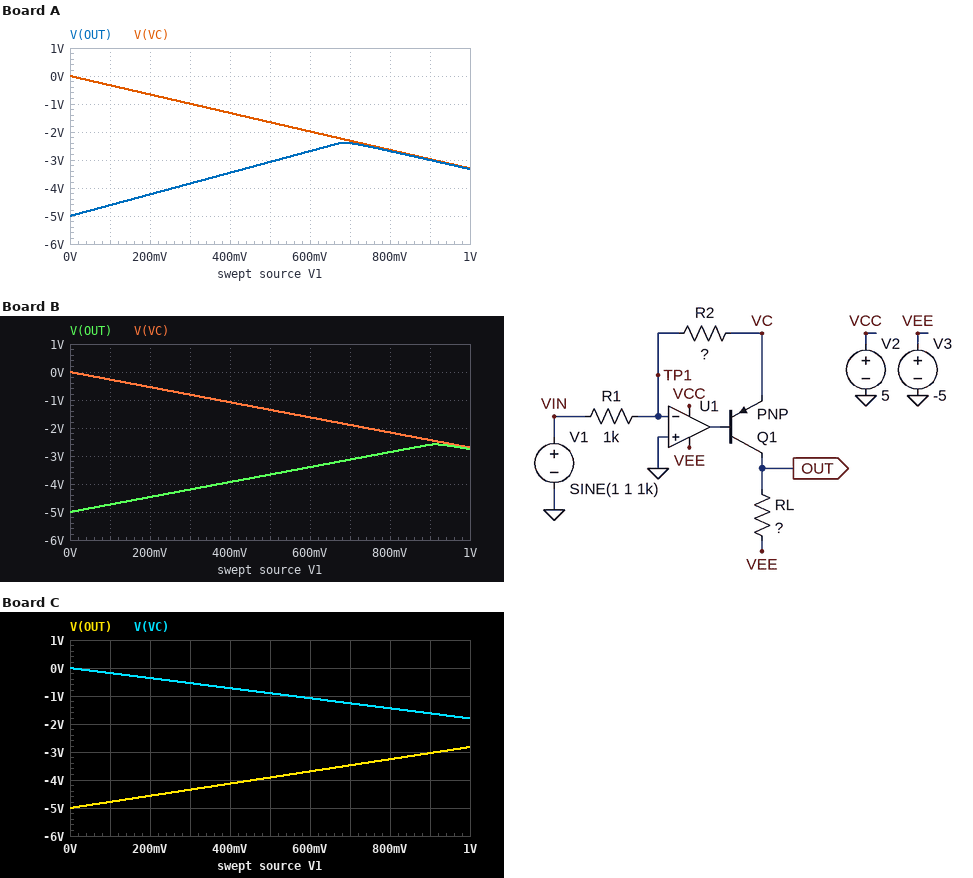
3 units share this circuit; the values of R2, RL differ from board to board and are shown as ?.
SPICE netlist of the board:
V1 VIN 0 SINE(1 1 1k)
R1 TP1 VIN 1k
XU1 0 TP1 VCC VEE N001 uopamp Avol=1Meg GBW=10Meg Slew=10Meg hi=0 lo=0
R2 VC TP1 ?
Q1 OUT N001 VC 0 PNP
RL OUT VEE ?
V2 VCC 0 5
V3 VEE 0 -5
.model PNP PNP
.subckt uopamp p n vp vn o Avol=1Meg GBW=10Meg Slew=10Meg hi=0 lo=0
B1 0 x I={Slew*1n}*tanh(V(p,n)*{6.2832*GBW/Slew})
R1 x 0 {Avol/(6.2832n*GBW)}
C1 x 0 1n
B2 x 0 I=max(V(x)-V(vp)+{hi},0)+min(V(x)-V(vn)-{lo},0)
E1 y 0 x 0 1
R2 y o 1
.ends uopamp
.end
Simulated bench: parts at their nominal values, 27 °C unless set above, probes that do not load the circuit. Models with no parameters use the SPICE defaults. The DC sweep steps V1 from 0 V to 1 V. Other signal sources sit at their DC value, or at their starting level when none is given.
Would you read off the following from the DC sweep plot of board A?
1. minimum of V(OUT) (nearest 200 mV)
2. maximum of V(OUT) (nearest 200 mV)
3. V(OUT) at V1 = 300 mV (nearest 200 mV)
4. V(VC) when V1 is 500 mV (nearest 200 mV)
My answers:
-5.0 V
-2.4 V
-3.8 V
-1.6 V
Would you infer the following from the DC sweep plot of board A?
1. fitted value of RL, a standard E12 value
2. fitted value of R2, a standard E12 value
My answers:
3.9 kΩ
3.3 kΩ
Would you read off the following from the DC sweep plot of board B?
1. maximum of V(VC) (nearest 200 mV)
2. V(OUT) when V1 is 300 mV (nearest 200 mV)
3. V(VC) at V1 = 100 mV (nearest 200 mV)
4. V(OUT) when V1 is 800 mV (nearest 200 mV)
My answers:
0 V
-4.2 V
-200 mV
-2.8 V
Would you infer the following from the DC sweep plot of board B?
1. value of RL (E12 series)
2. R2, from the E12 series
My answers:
2.7 kΩ
2.7 kΩ
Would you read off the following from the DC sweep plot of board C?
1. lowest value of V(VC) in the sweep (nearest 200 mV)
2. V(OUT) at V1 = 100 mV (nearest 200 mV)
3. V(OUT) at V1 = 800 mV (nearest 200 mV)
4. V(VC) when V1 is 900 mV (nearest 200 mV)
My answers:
-1.8 V
-4.8 V
-3.2 V
-1.6 V
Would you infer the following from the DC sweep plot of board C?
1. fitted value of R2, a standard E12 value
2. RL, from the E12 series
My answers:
1.8 kΩ
2.2 kΩ
